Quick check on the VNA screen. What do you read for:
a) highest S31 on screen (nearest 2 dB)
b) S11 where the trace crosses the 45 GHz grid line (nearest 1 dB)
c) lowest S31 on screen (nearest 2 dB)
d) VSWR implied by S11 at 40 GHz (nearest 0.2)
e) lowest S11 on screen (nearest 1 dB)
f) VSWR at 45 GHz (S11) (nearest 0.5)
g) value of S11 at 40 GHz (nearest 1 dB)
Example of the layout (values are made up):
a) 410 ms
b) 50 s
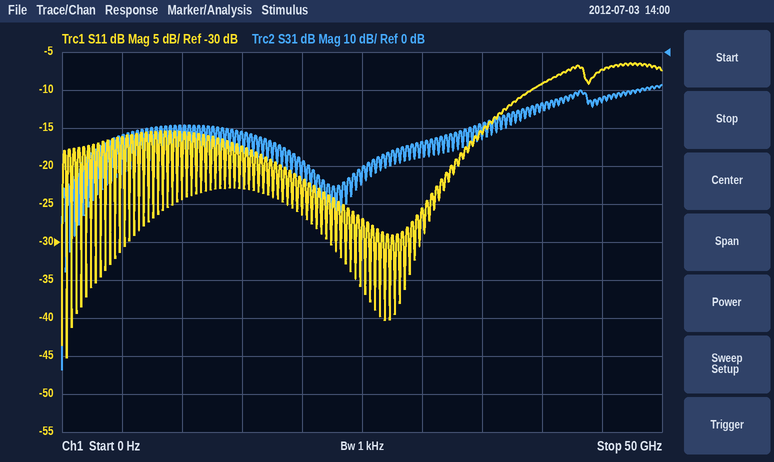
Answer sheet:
a) -8 dB
b) -7 dB
c) -84 dB
d) 2.0
e) -45 dB
f) 2.5
g) -9 dB
